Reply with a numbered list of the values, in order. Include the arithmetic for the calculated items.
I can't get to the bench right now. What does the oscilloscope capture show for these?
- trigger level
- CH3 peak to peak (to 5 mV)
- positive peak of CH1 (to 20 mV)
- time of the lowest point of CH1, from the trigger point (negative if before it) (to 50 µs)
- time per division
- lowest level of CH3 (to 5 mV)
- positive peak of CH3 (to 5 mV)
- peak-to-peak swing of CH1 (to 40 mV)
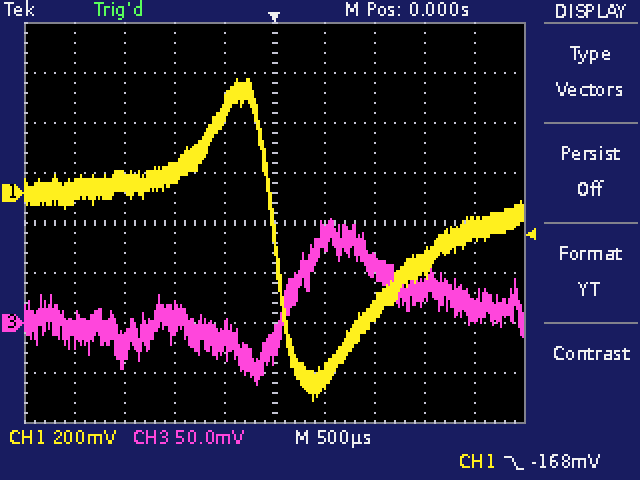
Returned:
1. -168 mV
2. 105 mV − (-60 mV) = 165 mV
3. 460 mV
4. +400 µs
5. 500 µs
6. -60 mV
7. 105 mV
8. 1.28 V
